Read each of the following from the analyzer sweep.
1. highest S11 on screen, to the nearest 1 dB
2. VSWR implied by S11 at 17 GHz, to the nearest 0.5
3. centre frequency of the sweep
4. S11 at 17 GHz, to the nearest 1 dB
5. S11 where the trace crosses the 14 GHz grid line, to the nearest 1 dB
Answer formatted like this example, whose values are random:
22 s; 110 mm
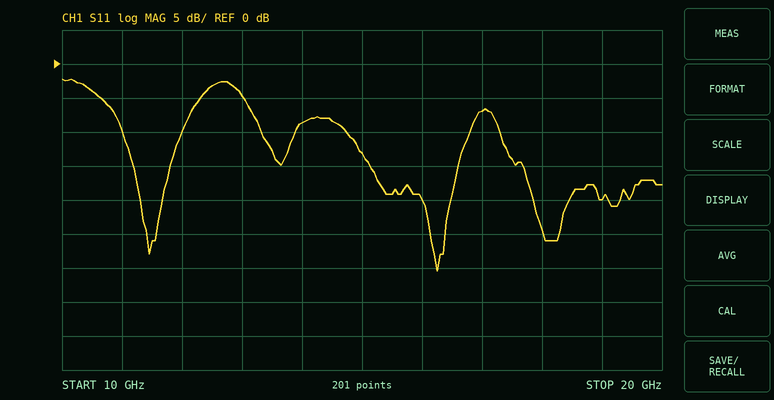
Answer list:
-2 dB; 2.5; 15 GHz; -7 dB; -9 dB
